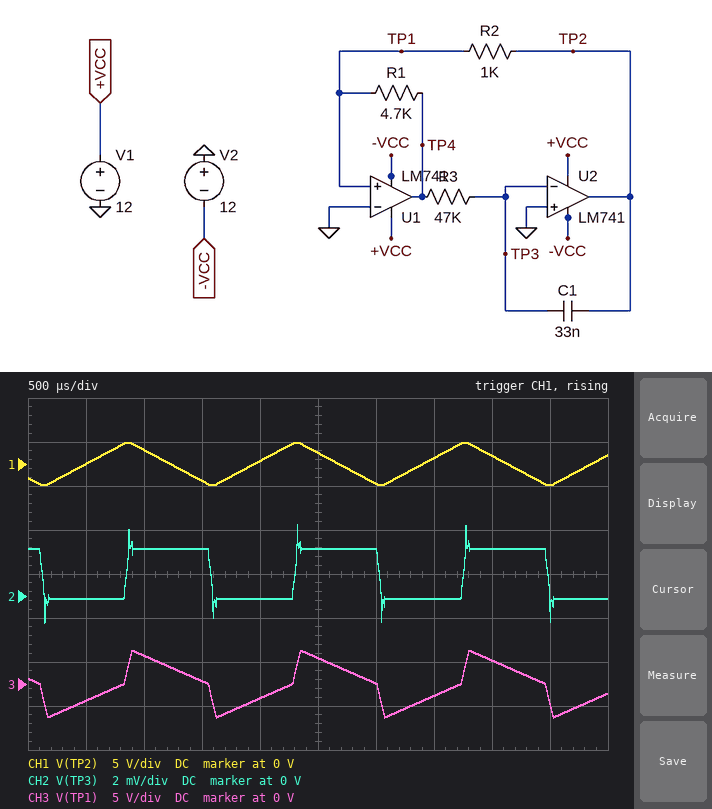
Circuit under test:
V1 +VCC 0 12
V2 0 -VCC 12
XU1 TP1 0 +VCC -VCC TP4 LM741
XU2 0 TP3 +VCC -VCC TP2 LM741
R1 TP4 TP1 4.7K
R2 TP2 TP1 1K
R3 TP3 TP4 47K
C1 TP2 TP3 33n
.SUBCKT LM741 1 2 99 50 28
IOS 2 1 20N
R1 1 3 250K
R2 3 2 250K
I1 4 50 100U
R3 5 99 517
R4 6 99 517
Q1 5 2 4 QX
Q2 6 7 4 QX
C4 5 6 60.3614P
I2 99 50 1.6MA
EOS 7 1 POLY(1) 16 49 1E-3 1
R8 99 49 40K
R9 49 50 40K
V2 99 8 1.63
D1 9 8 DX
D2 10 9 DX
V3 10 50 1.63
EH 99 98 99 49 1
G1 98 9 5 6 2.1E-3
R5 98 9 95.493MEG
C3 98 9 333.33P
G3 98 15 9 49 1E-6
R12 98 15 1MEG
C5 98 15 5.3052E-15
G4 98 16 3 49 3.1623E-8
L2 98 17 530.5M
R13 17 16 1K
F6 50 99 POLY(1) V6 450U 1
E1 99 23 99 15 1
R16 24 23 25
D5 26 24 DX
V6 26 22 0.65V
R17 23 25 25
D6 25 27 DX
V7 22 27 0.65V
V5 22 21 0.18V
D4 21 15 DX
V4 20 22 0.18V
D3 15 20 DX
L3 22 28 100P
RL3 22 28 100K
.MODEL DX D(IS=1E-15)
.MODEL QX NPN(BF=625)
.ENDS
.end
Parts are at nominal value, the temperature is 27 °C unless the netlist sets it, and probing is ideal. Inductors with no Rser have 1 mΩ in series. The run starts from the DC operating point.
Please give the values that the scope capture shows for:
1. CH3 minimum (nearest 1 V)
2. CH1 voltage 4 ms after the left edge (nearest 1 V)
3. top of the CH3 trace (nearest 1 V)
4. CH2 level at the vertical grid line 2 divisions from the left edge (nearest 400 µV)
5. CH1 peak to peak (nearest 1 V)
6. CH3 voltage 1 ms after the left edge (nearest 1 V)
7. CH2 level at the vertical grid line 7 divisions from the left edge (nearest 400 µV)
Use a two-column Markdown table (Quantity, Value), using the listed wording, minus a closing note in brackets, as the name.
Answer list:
| Quantity | Value |
|---|---|
| CH3 minimum | -4 V |
| CH1 voltage 4 ms after the left edge | 1 V |
| top of the CH3 trace | 4 V |
| CH2 level at the vertical grid line 2 divisions from the left edge | 2.0 mV |
| CH1 peak to peak | 5 V |
| CH3 voltage 1 ms after the left edge | 3 V |
| CH2 level at the vertical grid line 7 divisions from the left edge | 0 V |
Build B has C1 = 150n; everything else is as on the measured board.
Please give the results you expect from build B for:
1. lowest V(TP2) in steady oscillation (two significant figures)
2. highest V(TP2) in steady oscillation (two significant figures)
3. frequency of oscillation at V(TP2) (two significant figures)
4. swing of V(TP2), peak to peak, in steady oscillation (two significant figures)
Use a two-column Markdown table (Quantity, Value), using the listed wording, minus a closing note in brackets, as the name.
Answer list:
| Quantity | Value |
|---|---|
| lowest V(TP2) in steady oscillation | -2.3 V |
| highest V(TP2) in steady oscillation | 2.3 V |
| frequency of oscillation at V(TP2) | 160 Hz |
| swing of V(TP2), peak to peak, in steady oscillation | 4.7 V |
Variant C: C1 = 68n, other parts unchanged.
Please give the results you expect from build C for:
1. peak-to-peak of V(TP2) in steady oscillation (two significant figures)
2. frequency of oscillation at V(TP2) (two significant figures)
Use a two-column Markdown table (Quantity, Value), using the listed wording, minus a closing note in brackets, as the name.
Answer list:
| Quantity | Value |
|---|---|
| peak-to-peak of V(TP2) in steady oscillation | 4.7 V |
| frequency of oscillation at V(TP2) | 350 Hz |
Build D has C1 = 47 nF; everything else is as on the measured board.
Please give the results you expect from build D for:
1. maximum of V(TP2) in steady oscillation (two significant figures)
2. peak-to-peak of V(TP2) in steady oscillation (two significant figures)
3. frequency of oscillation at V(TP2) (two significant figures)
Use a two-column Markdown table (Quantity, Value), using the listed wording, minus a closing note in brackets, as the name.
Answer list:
| Quantity | Value |
|---|---|
| maximum of V(TP2) in steady oscillation | 2.4 V |
| peak-to-peak of V(TP2) in steady oscillation | 4.8 V |
| frequency of oscillation at V(TP2) | 500 Hz |
